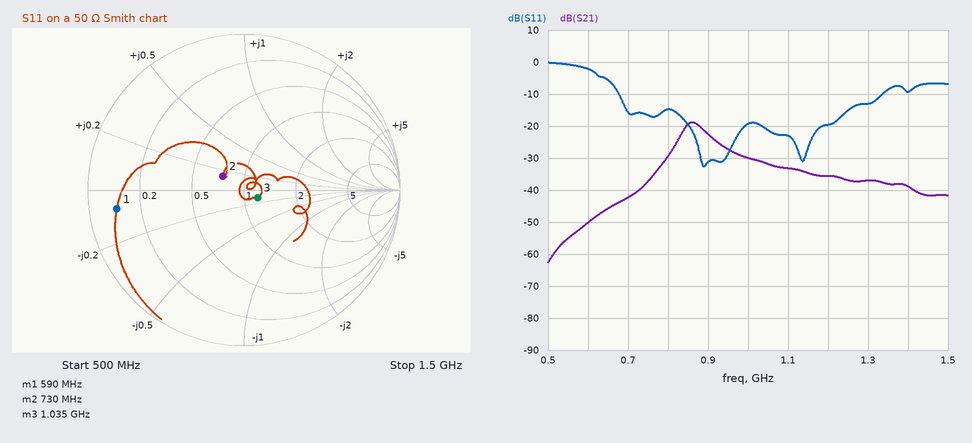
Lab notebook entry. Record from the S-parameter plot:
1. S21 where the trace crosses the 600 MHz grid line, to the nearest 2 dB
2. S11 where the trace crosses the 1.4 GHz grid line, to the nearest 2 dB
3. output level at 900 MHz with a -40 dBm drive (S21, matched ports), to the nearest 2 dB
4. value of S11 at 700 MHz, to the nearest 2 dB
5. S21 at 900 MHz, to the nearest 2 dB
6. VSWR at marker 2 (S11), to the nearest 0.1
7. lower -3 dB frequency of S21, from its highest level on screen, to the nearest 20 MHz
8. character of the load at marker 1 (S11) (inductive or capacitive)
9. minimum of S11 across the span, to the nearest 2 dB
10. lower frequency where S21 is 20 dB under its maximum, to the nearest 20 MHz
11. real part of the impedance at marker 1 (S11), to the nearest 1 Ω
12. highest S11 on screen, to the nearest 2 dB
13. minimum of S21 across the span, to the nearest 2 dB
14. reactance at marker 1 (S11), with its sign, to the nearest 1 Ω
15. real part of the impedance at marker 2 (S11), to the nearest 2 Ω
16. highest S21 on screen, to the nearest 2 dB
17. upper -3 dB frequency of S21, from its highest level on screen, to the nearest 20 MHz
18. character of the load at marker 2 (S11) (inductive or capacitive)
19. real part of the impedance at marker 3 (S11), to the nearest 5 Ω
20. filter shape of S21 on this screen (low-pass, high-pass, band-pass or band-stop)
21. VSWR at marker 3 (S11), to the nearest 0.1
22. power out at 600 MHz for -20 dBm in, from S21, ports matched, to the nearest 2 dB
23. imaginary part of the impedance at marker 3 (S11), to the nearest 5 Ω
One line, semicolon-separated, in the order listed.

-50 dB; -10 dB; -62 dBm; -16 dB; -22 dB; 1.4; 840 MHz; capacitive; -32 dB; 740 MHz; 5 Ω; 0 dB; -62 dB; -4 Ω; 38 Ω; -18 dB; 900 MHz; inductive; 60 Ω; band-pass; 1.2; -70 dBm; -5 Ω
